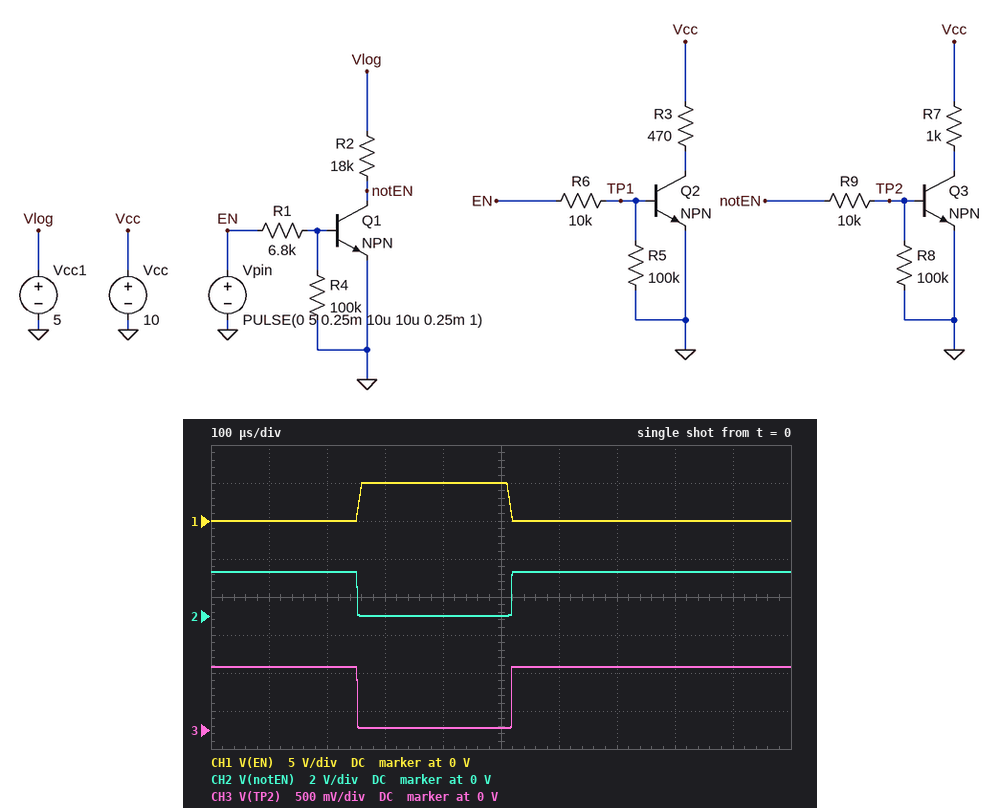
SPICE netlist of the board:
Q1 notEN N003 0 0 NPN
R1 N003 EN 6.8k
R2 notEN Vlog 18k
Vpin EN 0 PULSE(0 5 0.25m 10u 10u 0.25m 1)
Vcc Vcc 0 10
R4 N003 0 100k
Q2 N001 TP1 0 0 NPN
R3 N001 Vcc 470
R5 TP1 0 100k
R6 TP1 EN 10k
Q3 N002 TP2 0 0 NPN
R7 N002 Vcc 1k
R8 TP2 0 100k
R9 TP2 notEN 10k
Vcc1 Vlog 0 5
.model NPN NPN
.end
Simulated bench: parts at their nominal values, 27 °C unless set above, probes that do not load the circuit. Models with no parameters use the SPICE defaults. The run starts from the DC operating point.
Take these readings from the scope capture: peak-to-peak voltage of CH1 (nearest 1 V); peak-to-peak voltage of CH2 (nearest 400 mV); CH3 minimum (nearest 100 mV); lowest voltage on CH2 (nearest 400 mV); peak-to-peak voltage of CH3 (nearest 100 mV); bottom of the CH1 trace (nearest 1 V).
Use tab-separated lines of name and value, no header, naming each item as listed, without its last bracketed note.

peak-to-peak voltage of CH1	5 V
peak-to-peak voltage of CH2	2.4 V
CH3 minimum	0 V
lowest voltage on CH2	0 V
peak-to-peak voltage of CH3	800 mV
bottom of the CH1 trace	0 V
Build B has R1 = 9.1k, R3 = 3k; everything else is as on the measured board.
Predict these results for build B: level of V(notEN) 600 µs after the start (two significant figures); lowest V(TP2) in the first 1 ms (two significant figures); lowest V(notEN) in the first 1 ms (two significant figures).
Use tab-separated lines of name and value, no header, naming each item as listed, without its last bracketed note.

level of V(notEN) 600 µs after the start	2.3 V
lowest V(TP2) in the first 1 ms	23 mV
lowest V(notEN) in the first 1 ms	25 mV
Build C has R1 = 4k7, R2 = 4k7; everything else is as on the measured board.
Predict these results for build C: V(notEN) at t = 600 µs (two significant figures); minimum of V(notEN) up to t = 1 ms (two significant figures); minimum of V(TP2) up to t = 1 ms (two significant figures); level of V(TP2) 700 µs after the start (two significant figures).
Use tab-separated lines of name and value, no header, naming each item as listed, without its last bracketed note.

V(notEN) at t = 600 µs	3.7 V
minimum of V(notEN) up to t = 1 ms	30 mV
minimum of V(TP2) up to t = 1 ms	28 mV
level of V(TP2) 700 µs after the start	830 mV
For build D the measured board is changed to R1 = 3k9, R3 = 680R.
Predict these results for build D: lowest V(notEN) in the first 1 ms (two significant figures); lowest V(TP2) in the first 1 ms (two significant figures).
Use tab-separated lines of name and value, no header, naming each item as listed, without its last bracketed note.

lowest V(notEN) in the first 1 ms	21 mV
lowest V(TP2) in the first 1 ms	19 mV
